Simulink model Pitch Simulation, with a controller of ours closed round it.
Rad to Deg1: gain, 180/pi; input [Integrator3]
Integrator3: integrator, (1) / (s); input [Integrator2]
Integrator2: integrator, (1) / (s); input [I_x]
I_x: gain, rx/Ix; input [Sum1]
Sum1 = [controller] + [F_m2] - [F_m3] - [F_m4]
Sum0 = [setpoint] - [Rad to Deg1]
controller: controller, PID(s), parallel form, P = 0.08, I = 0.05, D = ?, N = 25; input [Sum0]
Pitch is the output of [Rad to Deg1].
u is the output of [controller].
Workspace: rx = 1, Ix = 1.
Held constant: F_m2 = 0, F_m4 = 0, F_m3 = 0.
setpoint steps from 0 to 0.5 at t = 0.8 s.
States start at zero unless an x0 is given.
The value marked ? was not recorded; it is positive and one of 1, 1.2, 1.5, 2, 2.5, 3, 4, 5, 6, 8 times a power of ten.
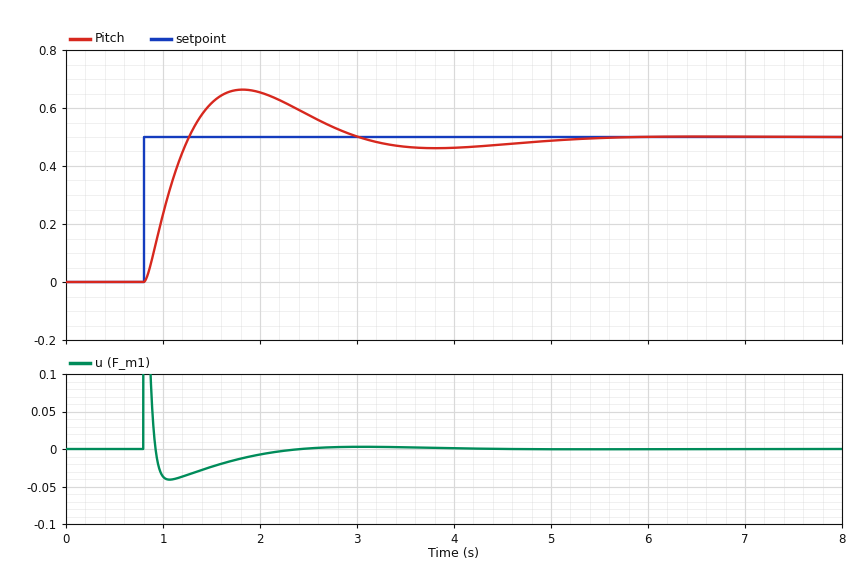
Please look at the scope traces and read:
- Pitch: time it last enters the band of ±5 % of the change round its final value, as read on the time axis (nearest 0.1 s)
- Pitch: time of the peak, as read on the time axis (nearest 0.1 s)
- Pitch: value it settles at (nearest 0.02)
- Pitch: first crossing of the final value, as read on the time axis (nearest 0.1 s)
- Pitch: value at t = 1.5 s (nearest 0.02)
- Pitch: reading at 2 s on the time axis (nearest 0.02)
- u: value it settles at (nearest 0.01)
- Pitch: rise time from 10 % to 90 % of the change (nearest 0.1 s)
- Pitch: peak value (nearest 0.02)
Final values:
4.5 s
1.8 s
0.50
1.3 s
0.62
0.66
0.00
0.3 s
0.66
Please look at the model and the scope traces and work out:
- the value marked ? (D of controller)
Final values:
0.05
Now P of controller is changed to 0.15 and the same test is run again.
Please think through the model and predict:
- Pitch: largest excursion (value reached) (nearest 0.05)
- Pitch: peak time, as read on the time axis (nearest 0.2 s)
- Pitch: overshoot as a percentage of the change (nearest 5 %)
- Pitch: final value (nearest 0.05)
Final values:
0.70
1.6 s
40 %
0.50
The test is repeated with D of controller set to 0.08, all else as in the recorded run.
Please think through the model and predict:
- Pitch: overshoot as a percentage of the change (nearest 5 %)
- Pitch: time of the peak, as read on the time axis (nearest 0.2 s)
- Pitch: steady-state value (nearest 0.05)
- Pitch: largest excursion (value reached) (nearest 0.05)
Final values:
20 %
1.6 s
0.50
0.60
